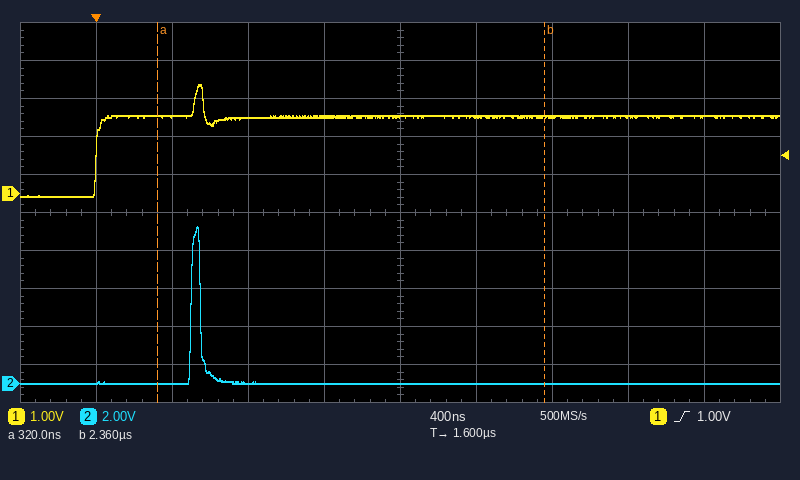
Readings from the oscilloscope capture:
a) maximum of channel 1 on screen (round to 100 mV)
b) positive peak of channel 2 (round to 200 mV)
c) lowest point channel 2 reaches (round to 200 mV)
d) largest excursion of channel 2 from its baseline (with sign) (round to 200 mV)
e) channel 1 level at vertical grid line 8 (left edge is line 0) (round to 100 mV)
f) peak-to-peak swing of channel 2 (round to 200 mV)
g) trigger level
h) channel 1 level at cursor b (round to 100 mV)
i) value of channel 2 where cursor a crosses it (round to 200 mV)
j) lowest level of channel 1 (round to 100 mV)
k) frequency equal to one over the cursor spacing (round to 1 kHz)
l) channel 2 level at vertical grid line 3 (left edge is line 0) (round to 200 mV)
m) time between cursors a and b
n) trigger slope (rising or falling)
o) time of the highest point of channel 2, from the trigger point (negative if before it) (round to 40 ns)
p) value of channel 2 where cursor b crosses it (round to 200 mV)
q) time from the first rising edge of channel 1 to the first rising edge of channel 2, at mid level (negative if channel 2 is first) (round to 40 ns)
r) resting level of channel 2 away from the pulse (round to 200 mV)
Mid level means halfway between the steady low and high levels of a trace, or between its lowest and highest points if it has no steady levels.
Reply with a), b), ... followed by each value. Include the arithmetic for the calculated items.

a) 2.9 V
b) 8.2 V
c) 0.0 V
d) 8.2 V − (0.0 V) = +8.2 V
e) 2.0 V
f) 8.2 V − (0.0 V) = 8.2 V
g) 1.00 V
h) 2.0 V
i) 0.0 V
j) -100 mV
k) 1 / 2.04 µs ≈ 490 kHz
l) 0.0 V
m) 2.36 µs − (320 ns) = 2.04 µs
n) rising
o) +520 ns
p) 0.0 V
q) +480 ns
r) 0.0 V
